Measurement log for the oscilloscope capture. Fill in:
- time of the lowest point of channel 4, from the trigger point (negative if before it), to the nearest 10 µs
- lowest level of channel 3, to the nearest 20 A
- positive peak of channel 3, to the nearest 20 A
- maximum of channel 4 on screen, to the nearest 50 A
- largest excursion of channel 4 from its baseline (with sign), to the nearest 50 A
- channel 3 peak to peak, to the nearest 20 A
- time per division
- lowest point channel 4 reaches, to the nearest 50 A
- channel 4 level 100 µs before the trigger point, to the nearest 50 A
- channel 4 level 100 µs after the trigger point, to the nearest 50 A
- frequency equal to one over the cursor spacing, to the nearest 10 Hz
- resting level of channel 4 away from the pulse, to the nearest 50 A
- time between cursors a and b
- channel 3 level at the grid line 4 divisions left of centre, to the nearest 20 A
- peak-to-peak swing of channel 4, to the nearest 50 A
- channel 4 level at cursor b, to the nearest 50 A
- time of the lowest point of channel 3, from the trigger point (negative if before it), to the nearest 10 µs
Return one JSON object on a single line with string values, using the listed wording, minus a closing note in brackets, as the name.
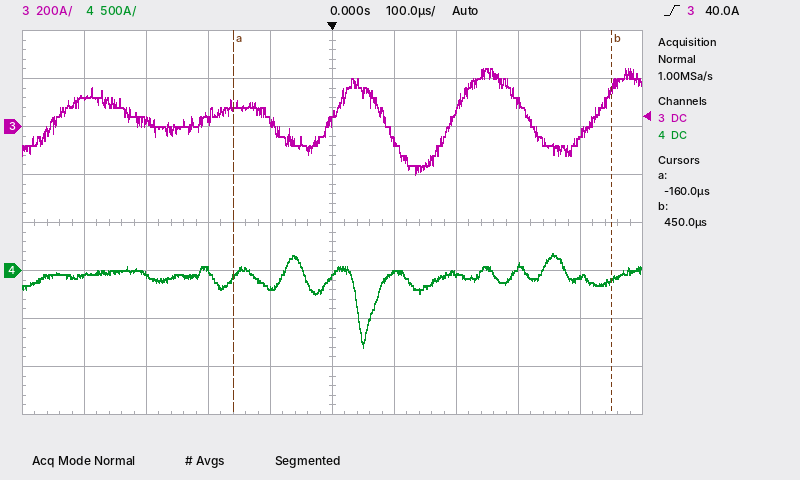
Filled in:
{"time of the lowest point of channel 4, from the trigger point (negative if before it), to the nearest 10 µs": "+50 µs", "lowest level of channel 3, to the nearest 20 A": "-200 A", "positive peak of channel 3, to the nearest 20 A": "240 A", "maximum of channel 4 on screen, to the nearest 50 A": "200 A", "largest excursion of channel 4 from its baseline (with sign), to the nearest 50 A": "-750 A", "channel 3 peak to peak, to the nearest 20 A": "440 A", "time per division": "100 µs", "lowest point channel 4 reaches, to the nearest 50 A": "-800 A", "channel 4 level 100 µs before the trigger point, to the nearest 50 A": "-200 A", "channel 4 level 100 µs after the trigger point, to the nearest 50 A": "0 A", "frequency equal to one over the cursor spacing, to the nearest 10 Hz": "1.64 kHz", "resting level of channel 4 away from the pulse, to the nearest 50 A": "-50 A", "time between cursors a and b": "610 µs", "channel 3 level at the grid line 4 divisions left of centre, to the nearest 20 A": "120 A", "peak-to-peak swing of channel 4, to the nearest 50 A": "1.00 kA", "channel 4 level at cursor b, to the nearest 50 A": "-100 A", "time of the lowest point of channel 3, from the trigger point (negative if before it), to the nearest 10 µs": "+140 µs"}
